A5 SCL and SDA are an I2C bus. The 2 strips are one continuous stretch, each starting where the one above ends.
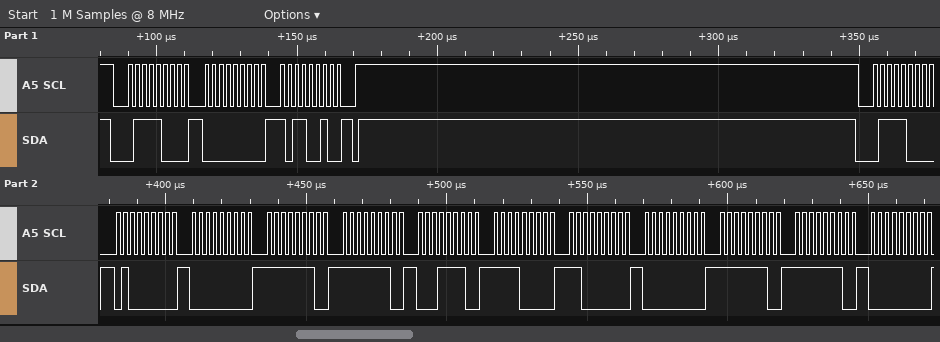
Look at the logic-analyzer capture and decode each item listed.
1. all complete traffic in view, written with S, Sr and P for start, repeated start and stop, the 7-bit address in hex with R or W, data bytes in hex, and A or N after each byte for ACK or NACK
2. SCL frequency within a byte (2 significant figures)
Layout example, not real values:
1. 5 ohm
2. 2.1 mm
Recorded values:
1. S 3CW A 00 A B2 A P S 3CW A 40 A 00 A FE A FE A 1E A F0 A C0 A 00 A FE A FE A 00 A
2. 400 kHz
